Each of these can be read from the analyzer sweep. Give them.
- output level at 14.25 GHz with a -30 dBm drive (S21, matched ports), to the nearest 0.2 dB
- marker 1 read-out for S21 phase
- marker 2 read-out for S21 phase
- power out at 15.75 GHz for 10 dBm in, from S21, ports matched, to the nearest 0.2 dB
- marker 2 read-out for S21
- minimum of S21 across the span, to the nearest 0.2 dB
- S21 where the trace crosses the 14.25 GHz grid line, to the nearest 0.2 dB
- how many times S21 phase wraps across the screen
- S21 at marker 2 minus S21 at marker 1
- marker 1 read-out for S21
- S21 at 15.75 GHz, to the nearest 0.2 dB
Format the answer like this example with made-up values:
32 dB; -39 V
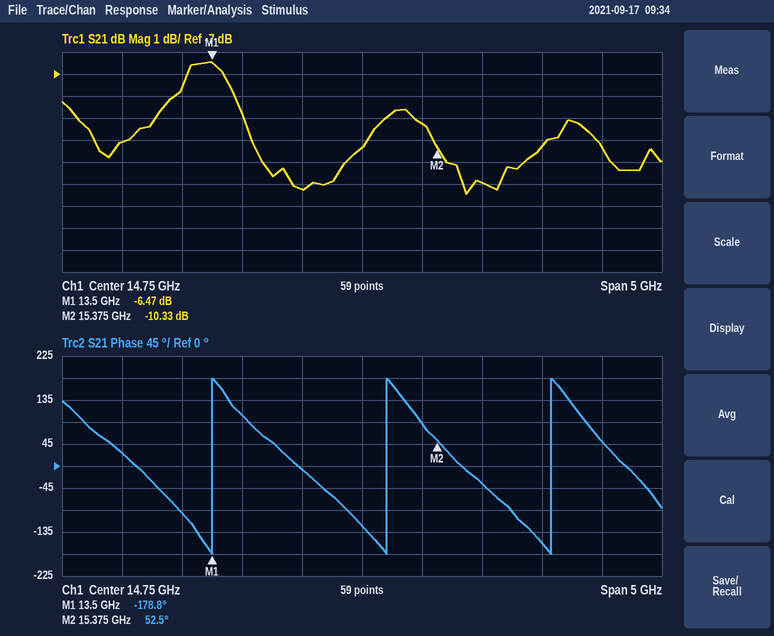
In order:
-42.2 dBm; -178.8°; 52.5°; -2.0 dBm; -10.33 dB; -12.4 dB; -12.2 dB; 3; -3.86 dB; -6.47 dB; -12.0 dB
